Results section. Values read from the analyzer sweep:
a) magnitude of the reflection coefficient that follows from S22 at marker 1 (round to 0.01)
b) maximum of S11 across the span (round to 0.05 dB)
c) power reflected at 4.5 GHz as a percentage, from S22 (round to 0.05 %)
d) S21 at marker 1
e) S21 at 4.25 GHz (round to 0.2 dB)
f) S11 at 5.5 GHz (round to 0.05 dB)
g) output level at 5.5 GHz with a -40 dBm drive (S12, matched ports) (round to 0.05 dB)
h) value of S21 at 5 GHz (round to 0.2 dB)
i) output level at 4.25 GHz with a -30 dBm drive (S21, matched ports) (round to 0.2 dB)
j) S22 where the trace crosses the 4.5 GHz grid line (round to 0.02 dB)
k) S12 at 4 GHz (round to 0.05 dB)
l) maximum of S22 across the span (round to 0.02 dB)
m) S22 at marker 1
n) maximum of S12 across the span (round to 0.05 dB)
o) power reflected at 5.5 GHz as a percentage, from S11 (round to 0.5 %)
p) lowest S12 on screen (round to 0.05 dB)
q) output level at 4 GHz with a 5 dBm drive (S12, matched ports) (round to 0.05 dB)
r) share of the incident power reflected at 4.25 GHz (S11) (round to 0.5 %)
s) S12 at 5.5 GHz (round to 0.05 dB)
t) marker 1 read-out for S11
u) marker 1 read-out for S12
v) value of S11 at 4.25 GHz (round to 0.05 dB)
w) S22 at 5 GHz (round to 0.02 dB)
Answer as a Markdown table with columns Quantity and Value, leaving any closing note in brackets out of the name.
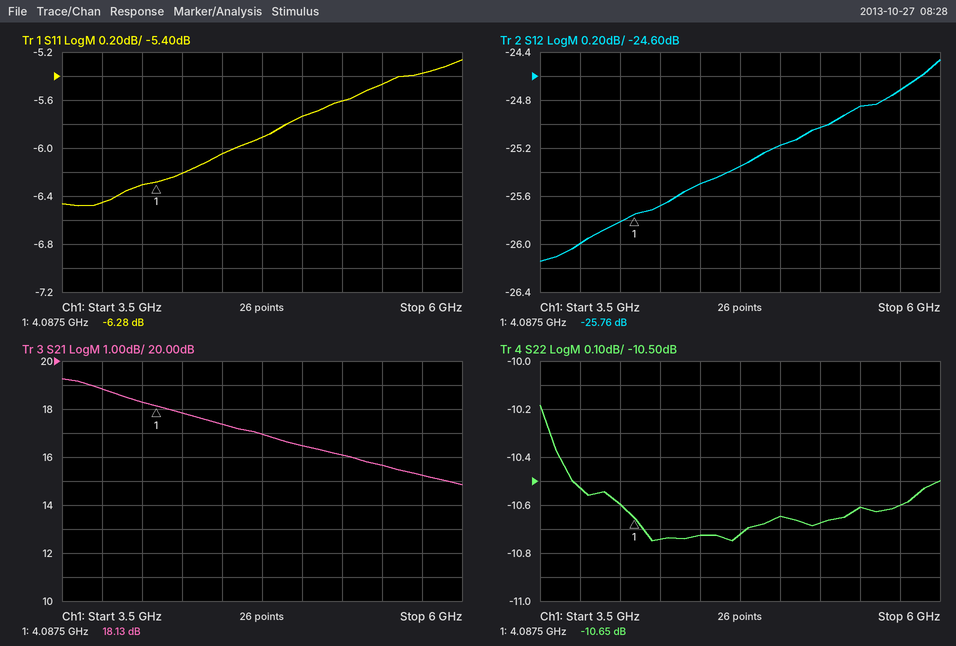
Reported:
| Quantity | Value |
|---|---|
| magnitude of the reflection coefficient that follows from S22 at marker 1 | 0.29 |
| maximum of S11 across the span | -5.25 dB |
| power reflected at 4.5 GHz as a percentage, from S22 | 8.45 % |
| S21 at marker 1 | 18.13 dB |
| S21 at 4.25 GHz | 17.8 dB |
| S11 at 5.5 GHz | -5.45 dB |
| output level at 5.5 GHz with a -40 dBm drive (S12, matched ports) | -64.85 dBm |
| value of S21 at 5 GHz | 16.4 dB |
| output level at 4.25 GHz with a -30 dBm drive (S21, matched ports) | -12.2 dBm |
| S22 where the trace crosses the 4.5 GHz grid line | -10.72 dB |
| S12 at 4 GHz | -25.80 dB |
| maximum of S22 across the span | -10.18 dB |
| S22 at marker 1 | -10.65 dB |
| maximum of S12 across the span | -24.45 dB |
| power reflected at 5.5 GHz as a percentage, from S11 | 28.5 % |
| lowest S12 on screen | -26.15 dB |
| output level at 4 GHz with a 5 dBm drive (S12, matched ports) | -20.80 dBm |
| share of the incident power reflected at 4.25 GHz (S11) | 24.0 % |
| S12 at 5.5 GHz | -24.85 dB |
| marker 1 read-out for S11 | -6.28 dB |
| marker 1 read-out for S12 | -25.76 dB |
| value of S11 at 4.25 GHz | -6.20 dB |
| S22 at 5 GHz | -10.64 dB |
